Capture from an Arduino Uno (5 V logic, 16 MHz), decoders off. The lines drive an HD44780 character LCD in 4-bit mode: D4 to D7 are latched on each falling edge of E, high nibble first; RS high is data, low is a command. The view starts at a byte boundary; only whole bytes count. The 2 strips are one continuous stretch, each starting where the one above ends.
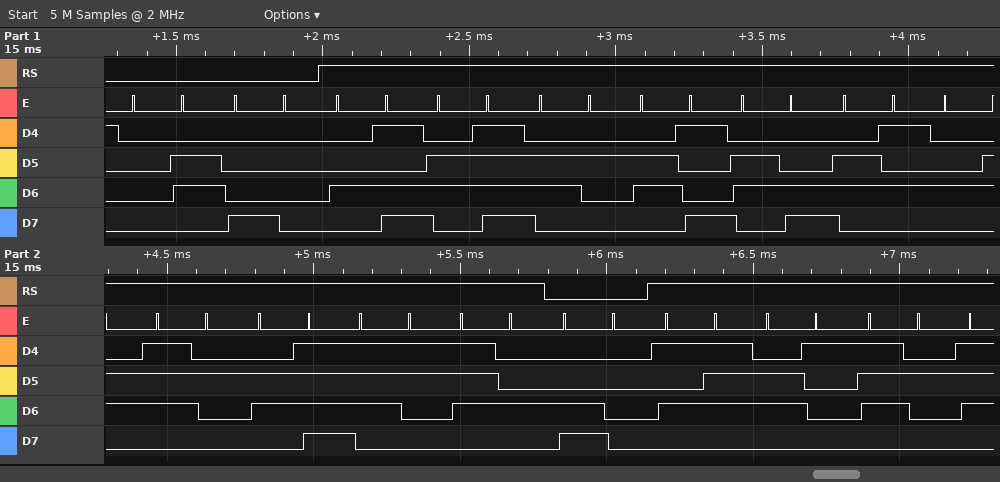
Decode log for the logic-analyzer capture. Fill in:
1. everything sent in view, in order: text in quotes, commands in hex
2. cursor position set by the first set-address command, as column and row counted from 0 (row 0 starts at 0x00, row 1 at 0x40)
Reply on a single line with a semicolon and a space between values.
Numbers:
0x06 0x80 "MobileFrost" 0xC0 "War"; column 0, row 0
